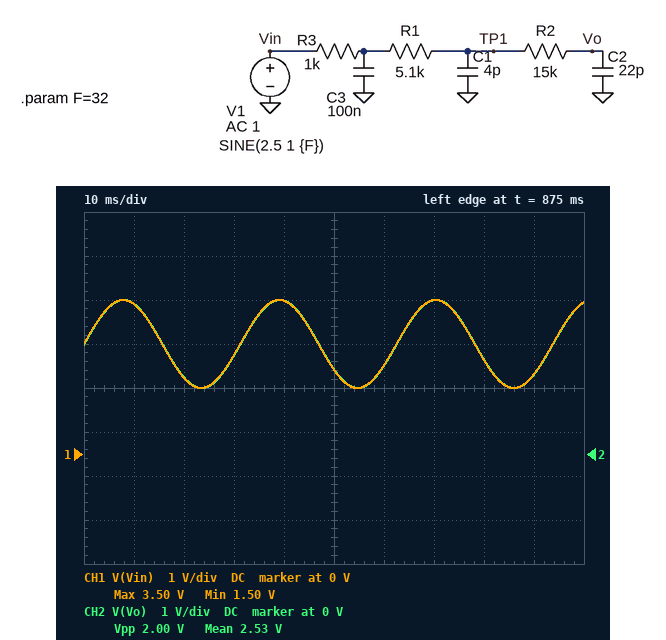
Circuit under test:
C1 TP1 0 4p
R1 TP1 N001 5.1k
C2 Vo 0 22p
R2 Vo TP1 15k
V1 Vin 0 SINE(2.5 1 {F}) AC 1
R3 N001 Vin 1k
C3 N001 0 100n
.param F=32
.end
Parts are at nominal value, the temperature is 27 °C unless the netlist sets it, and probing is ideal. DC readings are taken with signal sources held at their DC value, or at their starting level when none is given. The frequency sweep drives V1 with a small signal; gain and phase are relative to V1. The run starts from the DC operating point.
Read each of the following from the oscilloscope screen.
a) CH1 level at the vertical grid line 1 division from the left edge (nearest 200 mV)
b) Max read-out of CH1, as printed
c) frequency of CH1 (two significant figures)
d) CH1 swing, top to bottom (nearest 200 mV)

3.4 V
3.50 V
32 Hz
2.0 V
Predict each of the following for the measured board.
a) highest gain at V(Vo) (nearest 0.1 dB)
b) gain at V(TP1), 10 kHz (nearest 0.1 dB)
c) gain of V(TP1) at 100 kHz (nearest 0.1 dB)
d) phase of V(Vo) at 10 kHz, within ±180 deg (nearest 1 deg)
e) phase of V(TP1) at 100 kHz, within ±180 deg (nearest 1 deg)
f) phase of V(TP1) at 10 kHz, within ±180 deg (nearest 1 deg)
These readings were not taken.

0 dB
-16.1 dB
-36.1 dB
-83 deg
-94 deg
-81 deg
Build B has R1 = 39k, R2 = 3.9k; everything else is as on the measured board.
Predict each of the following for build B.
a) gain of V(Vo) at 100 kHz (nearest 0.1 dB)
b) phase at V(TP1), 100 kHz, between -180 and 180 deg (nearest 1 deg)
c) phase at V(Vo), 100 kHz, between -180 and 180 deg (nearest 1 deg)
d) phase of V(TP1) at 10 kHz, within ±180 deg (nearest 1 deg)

-37.6 dB
-121 deg
-124 deg
-85 deg
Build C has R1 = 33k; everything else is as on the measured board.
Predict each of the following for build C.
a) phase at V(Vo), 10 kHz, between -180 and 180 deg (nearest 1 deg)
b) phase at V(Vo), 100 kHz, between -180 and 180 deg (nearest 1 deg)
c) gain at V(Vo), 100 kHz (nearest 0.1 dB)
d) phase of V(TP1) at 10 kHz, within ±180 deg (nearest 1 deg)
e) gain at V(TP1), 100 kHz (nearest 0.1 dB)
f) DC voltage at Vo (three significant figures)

-85 deg
-126 deg
-37.8 dB
-84 deg
-37.6 dB
2.50 V
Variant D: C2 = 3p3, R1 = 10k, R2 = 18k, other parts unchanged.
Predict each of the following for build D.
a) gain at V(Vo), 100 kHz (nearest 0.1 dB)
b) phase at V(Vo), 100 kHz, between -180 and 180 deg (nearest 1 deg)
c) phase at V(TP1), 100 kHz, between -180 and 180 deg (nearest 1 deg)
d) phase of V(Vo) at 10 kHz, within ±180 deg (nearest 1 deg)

-36.0 dB
-94 deg
-92 deg
-81 deg
